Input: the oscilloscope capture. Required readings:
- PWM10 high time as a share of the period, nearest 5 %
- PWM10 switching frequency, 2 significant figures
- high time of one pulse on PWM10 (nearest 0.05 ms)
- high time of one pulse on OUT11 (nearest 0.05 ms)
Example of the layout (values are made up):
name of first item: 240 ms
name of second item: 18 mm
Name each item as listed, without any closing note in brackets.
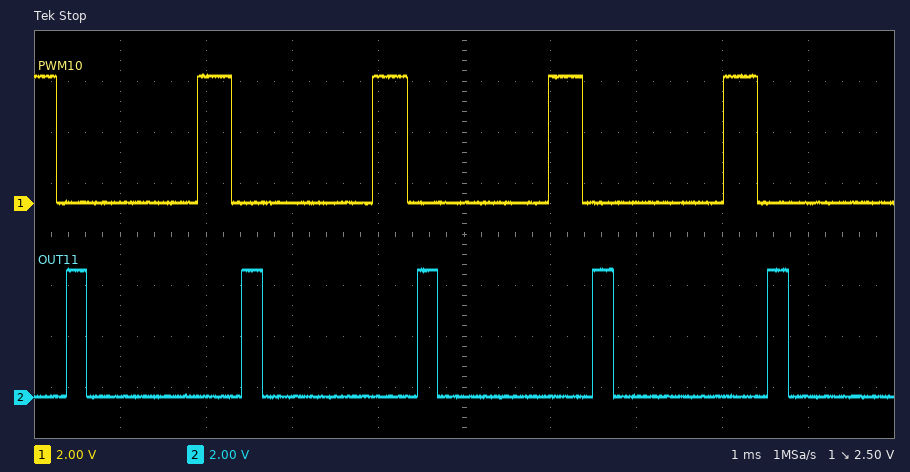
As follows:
PWM10 high time as a share of the period, nearest 5 %: 20 %
PWM10 switching frequency, 2 significant figures: 490 Hz
high time of one pulse on PWM10: 0.40 ms
high time of one pulse on OUT11: 0.25 ms
